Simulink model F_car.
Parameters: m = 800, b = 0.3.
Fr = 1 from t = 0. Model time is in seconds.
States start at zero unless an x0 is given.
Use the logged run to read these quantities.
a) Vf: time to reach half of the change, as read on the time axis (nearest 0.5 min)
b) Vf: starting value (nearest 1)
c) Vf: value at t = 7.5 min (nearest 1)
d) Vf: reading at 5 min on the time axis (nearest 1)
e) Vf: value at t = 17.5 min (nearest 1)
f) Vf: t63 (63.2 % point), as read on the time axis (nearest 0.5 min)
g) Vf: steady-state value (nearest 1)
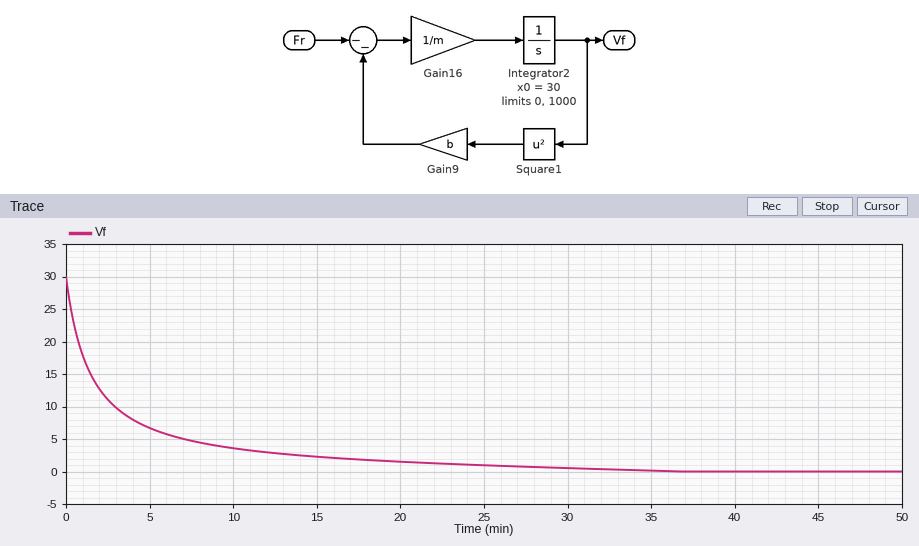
1.5 min
30
5
7
2
2.5 min
0
